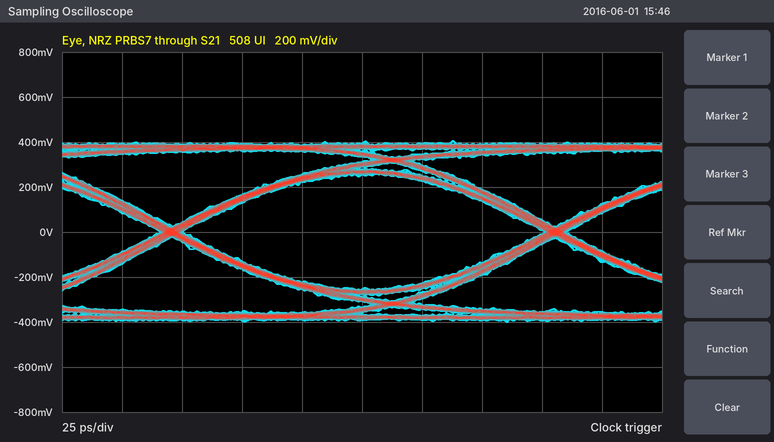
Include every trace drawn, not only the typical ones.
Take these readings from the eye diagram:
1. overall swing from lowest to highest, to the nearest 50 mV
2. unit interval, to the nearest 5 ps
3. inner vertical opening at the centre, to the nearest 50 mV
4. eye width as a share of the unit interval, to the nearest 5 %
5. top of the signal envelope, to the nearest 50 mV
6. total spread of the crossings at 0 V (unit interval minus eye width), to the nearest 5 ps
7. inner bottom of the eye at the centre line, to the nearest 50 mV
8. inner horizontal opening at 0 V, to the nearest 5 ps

800 mV
160 ps
500 mV
95 %
400 mV
10 ps
-250 mV
150 ps
